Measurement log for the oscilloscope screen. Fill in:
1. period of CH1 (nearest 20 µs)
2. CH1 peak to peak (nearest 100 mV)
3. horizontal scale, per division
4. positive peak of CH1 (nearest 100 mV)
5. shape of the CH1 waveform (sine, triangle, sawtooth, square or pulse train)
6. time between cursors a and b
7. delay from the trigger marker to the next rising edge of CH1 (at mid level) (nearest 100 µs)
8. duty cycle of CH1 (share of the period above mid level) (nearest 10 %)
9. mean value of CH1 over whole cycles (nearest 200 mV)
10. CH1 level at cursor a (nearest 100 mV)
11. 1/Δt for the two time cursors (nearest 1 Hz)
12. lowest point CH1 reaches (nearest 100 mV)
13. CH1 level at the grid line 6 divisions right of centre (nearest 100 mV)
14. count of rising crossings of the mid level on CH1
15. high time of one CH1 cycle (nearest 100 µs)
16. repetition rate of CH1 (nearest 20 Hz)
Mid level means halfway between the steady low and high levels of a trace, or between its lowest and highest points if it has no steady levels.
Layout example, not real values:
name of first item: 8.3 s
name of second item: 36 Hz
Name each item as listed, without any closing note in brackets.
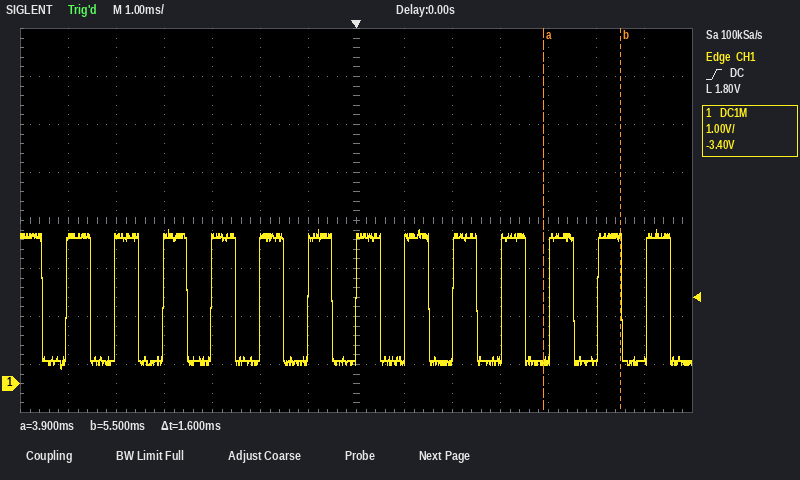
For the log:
period of CH1: 1.00 ms
CH1 peak to peak: 2.9 V
horizontal scale, per division: 1 ms
positive peak of CH1: 3.2 V
shape of the CH1 waveform: square
time between cursors a and b: 1.6 ms
delay from the trigger marker to the next rising edge of CH1 (at mid level): 1.0 ms
duty cycle of CH1 (share of the period above mid level): 50 %
mean value of CH1 over whole cycles: 1.8 V
CH1 level at cursor a: 500 mV
1/Δt for the two time cursors: 625 Hz
lowest point CH1 reaches: 300 mV
CH1 level at the grid line 6 divisions right of centre: 500 mV
count of rising crossings of the mid level on CH1: 13
high time of one CH1 cycle: 500 µs
repetition rate of CH1: 1.00 kHz
